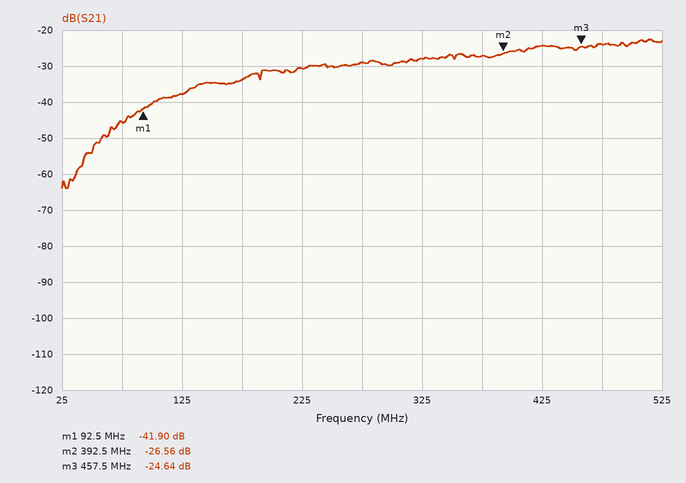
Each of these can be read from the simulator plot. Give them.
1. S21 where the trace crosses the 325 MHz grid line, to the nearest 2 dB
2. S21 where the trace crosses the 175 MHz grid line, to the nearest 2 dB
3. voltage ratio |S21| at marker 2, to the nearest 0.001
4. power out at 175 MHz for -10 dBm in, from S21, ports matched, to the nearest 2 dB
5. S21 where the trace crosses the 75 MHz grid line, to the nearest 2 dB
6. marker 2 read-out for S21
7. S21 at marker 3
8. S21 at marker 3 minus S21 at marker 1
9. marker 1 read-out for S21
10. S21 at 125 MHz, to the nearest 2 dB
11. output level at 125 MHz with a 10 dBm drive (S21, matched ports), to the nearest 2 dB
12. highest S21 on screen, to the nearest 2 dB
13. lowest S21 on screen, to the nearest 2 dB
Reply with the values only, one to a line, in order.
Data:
-28 dB
-34 dB
0.047
-44 dBm
-46 dB
-26.56 dB
-24.64 dB
17.26 dB
-41.90 dB
-38 dB
-28 dBm
-22 dB
-64 dB
